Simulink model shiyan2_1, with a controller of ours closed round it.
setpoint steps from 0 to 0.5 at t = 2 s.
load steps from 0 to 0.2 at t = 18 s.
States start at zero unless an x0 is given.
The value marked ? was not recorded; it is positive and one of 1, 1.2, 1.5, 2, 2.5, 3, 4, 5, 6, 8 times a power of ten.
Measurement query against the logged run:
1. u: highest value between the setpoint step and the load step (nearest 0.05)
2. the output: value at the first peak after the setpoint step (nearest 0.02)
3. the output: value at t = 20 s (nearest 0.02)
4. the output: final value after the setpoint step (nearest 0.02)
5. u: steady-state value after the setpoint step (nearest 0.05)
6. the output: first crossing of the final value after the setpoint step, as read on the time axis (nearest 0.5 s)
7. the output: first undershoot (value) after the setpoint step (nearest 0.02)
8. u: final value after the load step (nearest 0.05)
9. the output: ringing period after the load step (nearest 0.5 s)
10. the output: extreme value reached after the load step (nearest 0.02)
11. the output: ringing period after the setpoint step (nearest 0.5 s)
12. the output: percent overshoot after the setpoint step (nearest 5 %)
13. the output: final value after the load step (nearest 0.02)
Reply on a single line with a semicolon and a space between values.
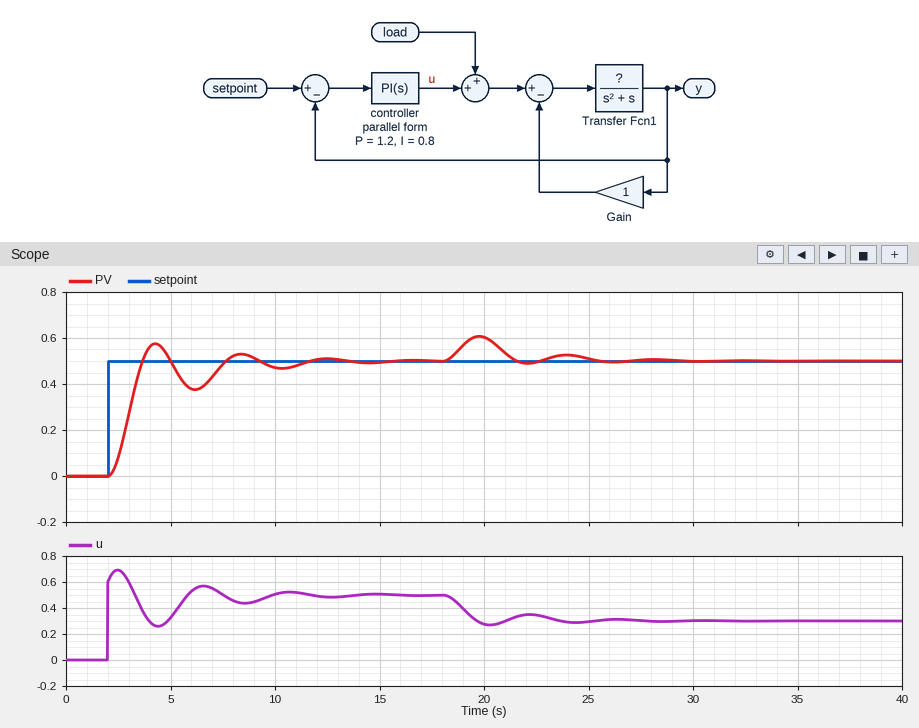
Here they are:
0.70; 0.58; 0.60; 0.50; 0.50; 3.5 s; 0.38; 0.30; 4.0 s; 0.60; 4.0 s; 15 %; 0.50
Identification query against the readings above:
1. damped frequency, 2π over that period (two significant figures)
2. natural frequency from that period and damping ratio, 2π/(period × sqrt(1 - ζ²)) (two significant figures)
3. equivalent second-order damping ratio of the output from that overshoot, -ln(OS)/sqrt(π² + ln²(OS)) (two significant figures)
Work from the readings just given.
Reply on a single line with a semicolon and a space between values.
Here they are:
1.6 rad/s; 1.8 rad/s; 0.52
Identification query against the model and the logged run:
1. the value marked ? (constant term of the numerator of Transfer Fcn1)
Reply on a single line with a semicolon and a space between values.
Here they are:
1.2
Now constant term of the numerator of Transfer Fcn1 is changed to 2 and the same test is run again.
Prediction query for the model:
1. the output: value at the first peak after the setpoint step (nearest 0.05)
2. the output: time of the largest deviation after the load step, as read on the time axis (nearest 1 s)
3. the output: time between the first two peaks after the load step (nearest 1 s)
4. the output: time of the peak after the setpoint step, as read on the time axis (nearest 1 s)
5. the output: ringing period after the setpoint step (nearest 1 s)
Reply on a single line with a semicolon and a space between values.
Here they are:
0.55; 19 s; 3 s; 4 s; 3 s
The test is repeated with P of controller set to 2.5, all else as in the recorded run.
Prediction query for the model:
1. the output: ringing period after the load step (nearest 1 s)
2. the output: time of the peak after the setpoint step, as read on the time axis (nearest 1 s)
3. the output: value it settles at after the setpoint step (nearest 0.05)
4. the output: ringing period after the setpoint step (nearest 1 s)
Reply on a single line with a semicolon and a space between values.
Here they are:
3 s; 4 s; 0.50; 3 s
